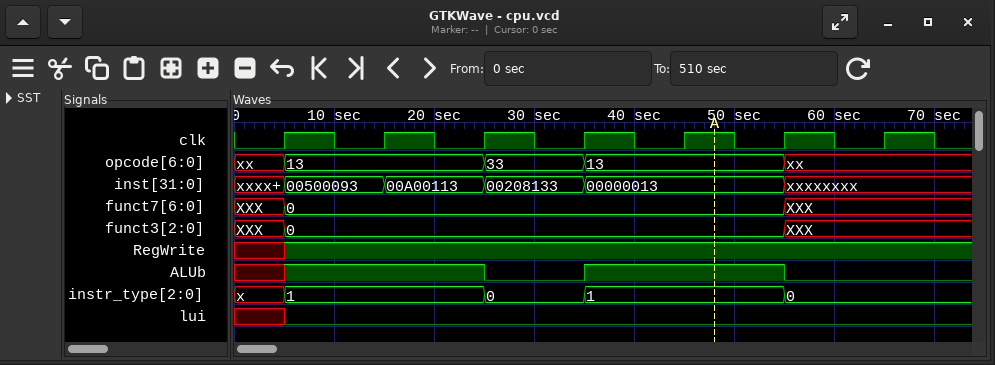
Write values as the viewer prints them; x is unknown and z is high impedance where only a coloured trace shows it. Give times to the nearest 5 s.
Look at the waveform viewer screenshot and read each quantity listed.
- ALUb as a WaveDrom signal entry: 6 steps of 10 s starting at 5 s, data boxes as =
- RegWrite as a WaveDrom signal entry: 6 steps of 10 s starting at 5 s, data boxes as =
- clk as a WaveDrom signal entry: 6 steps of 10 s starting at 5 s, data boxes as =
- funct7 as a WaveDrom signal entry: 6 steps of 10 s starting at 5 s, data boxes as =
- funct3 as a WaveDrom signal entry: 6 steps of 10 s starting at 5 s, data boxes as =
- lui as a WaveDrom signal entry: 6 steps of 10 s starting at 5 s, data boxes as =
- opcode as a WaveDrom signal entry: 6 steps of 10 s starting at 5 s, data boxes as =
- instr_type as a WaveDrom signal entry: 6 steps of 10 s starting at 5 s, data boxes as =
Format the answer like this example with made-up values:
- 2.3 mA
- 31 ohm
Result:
- {name: 'ALUb', wave: '1.01.0'}
- {name: 'RegWrite', wave: '1.....'}
- {name: 'clk', wave: 'p.....'}
- {name: 'funct7', wave: '=....x', data: '0'}
- {name: 'funct3', wave: '=....x', data: '0'}
- {name: 'lui', wave: '0.....'}
- {name: 'opcode', wave: '=.==.x', data: '13 33 13'}
- {name: 'instr_type', wave: '=.==.=', data: '1 0 1 0'}
